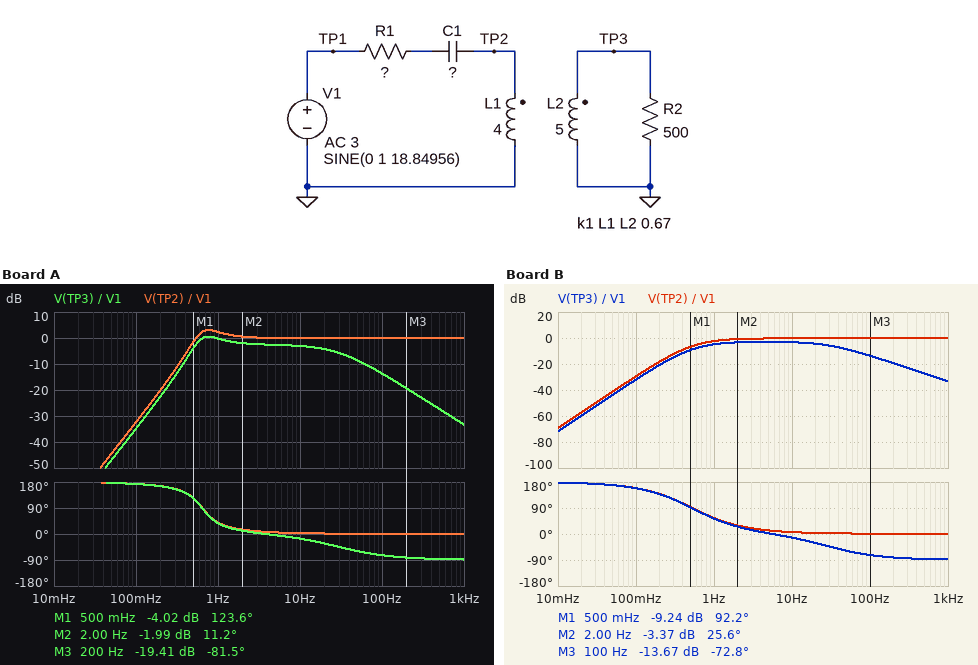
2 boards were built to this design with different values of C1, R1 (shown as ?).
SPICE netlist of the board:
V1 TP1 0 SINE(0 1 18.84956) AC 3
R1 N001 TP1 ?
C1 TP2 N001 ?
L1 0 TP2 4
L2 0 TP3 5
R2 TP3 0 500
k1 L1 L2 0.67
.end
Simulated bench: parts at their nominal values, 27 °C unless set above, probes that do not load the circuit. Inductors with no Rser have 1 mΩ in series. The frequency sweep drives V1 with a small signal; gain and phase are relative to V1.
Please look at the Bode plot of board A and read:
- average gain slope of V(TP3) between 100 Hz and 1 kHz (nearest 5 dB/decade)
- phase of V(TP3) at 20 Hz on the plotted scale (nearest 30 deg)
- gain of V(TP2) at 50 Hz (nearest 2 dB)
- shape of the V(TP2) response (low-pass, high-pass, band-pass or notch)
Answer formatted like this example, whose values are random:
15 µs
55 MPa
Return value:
-20 dB/decade
-30 deg
0 dB
high-pass
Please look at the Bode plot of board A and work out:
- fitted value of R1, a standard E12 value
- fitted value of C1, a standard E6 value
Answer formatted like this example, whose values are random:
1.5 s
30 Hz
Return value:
12 Ω
15 mF
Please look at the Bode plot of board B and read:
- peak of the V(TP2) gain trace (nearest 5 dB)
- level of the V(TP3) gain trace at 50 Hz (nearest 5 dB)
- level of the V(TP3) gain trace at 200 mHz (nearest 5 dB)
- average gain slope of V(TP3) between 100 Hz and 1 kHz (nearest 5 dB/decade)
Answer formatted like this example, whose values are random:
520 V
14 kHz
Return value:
0 dB
-10 dB
-20 dB
-20 dB/decade
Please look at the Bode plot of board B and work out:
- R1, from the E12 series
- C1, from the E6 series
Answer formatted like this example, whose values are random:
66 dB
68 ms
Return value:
27 Ω
22 mF
